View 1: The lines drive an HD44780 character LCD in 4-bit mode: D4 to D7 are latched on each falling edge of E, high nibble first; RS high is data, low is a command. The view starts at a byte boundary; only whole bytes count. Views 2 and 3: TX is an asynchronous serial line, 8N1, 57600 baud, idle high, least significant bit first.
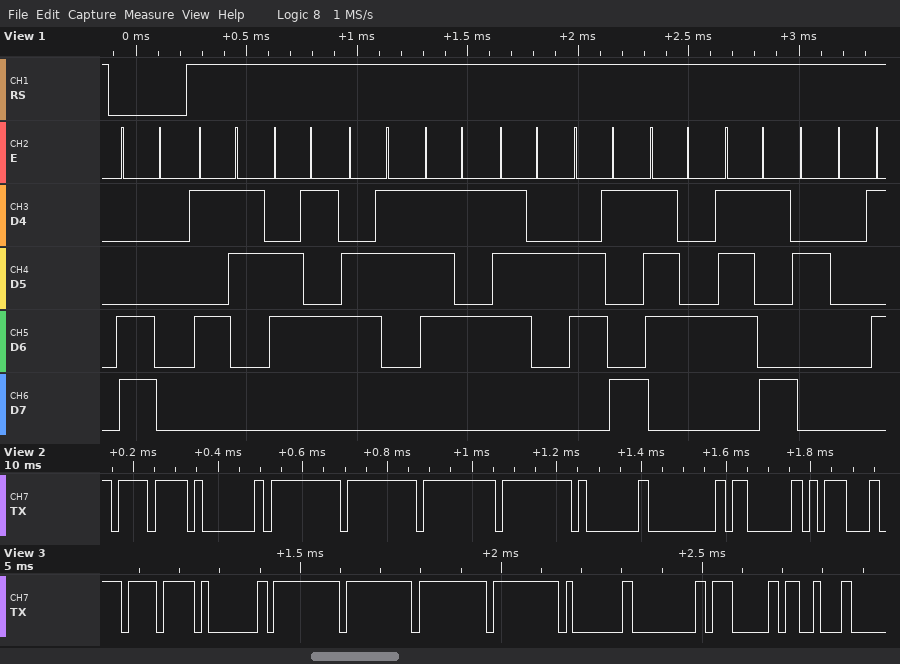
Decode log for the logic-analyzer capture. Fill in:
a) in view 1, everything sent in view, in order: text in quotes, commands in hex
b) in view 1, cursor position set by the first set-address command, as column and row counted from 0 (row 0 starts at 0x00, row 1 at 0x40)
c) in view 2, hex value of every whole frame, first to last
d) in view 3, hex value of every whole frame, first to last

0xC0 "Security "
column 0, row 1
0xEF 0x01 0xFF 0xFF 0xFF 0xFF 0x01 0x00 0x03 0x1D
EF 01 FF FF FF FF 01 00 07 13
